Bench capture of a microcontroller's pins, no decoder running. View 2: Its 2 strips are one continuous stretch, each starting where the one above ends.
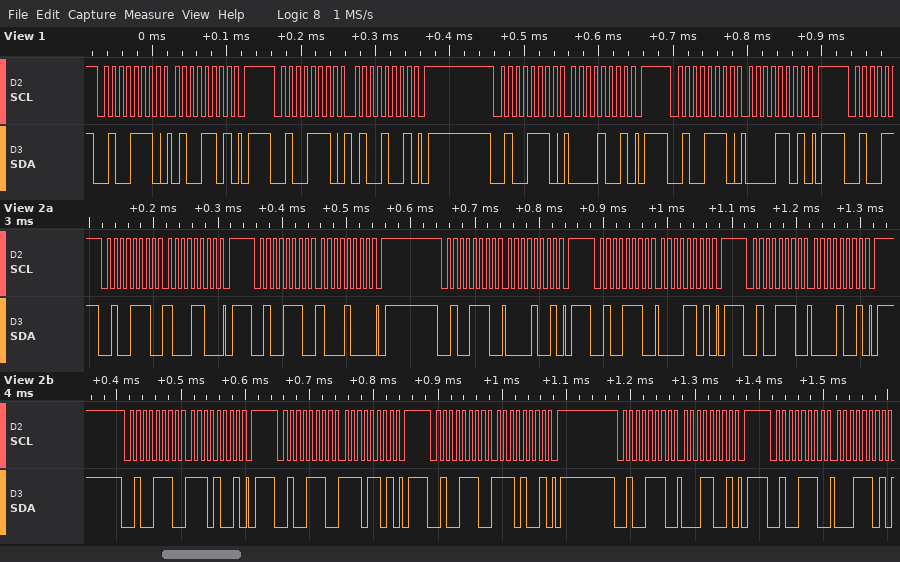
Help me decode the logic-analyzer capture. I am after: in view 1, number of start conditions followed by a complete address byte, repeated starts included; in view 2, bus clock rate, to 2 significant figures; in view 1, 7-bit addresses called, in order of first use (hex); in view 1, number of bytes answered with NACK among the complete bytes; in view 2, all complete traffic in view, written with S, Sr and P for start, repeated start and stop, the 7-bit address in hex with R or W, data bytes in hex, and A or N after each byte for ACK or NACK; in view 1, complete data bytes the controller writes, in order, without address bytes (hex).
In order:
4
100 kHz
0x27
0
S 27W A 8C A P S 27W A 88 A P S 27W A 09 A P S 27W A 0D A P S 27W A 09 A P S 27W A E9 A P S 27W A ED A P S 27W A E9 A P S 27W A 19 A P S 27W A 1D A
4D 49 09 0D
